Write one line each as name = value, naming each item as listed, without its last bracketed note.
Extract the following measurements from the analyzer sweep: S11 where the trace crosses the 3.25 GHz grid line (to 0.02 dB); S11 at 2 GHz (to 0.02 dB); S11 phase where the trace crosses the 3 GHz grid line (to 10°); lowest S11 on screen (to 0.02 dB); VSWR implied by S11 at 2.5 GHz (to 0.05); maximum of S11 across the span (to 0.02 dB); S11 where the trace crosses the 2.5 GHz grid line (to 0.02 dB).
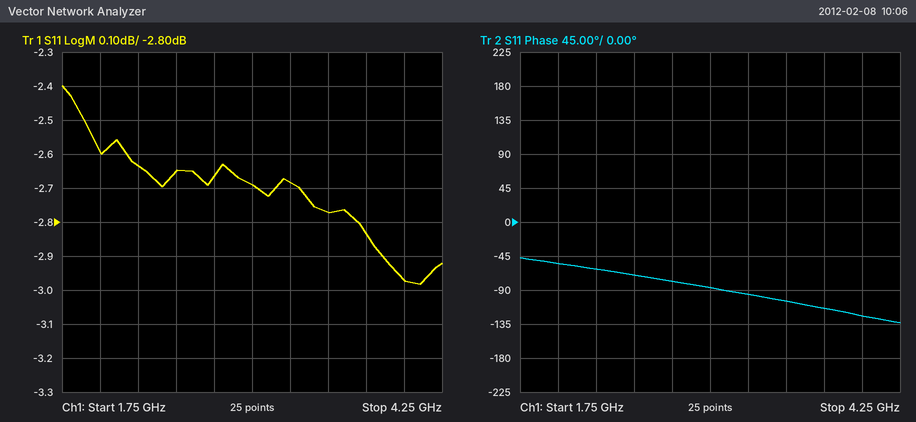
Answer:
S11 where the trace crosses the 3.25 GHz grid line = -2.68 dB
S11 at 2 GHz = -2.60 dB
S11 phase where the trace crosses the 3 GHz grid line = -90°
lowest S11 on screen = -2.98 dB
VSWR implied by S11 at 2.5 GHz = 6.60
maximum of S11 across the span = -2.40 dB
S11 where the trace crosses the 2.5 GHz grid line = -2.66 dB
